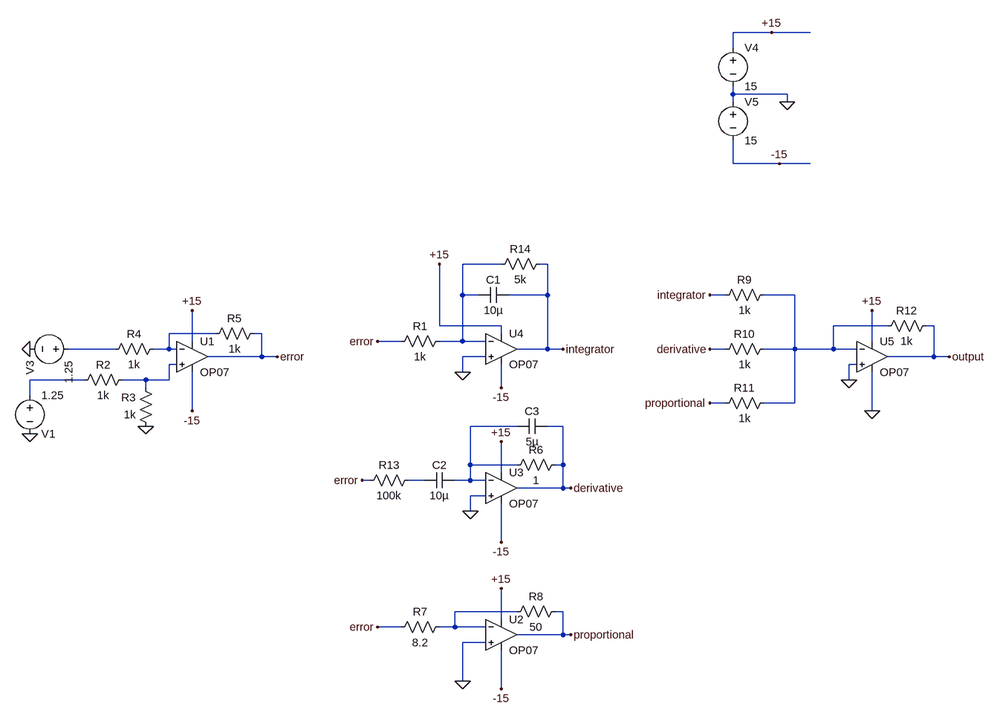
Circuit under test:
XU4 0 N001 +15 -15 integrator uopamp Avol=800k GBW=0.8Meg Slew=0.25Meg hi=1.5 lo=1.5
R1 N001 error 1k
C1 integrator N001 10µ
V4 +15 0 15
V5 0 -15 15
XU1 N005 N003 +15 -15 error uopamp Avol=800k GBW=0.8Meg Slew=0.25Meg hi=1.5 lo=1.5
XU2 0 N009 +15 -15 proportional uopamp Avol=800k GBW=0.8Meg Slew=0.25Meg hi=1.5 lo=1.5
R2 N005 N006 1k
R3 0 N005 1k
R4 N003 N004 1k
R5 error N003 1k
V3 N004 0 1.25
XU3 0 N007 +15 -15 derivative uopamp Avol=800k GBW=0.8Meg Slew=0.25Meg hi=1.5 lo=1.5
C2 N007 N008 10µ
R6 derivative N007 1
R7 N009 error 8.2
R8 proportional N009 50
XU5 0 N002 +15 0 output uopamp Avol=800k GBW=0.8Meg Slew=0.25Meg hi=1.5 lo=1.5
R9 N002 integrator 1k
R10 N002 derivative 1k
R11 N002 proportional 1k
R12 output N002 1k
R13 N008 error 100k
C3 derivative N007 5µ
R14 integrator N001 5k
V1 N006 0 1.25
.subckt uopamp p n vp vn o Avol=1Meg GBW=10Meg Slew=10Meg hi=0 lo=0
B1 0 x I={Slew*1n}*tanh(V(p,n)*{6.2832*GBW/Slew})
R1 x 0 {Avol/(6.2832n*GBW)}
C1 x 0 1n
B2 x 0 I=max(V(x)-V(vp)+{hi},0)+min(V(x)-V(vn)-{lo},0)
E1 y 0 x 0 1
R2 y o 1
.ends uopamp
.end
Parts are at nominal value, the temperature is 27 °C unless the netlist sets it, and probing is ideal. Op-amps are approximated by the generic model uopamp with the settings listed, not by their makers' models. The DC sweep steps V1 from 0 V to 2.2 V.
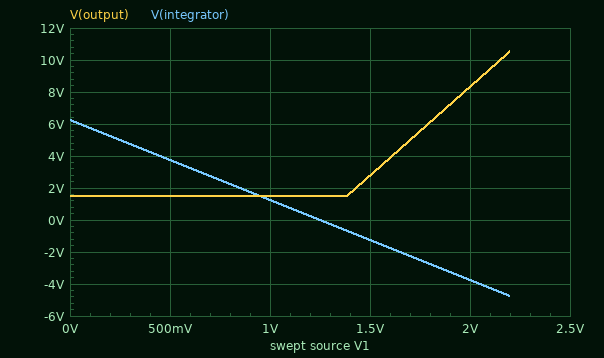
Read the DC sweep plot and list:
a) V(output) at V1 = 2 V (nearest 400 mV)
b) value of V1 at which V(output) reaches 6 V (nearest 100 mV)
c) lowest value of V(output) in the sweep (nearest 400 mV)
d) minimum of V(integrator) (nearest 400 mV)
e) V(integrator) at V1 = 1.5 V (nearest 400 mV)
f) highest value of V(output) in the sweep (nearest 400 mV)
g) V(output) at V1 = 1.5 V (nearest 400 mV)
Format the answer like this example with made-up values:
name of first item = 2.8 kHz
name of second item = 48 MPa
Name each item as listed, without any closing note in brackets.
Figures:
V(output) at V1 = 2 V = 8.4 V
value of V1 at which V(output) reaches 6 V = 1.8 V
lowest value of V(output) in the sweep = 1.6 V
minimum of V(integrator) = -4.8 V
V(integrator) at V1 = 1.5 V = -1.2 V
highest value of V(output) in the sweep = 10.4 V
V(output) at V1 = 1.5 V = 2.8 V
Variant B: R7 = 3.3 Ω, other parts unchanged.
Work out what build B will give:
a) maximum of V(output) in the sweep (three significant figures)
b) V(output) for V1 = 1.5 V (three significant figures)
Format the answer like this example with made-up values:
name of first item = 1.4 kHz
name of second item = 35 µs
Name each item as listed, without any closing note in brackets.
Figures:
maximum of V(output) in the sweep = 13.5 V
V(output) for V1 = 1.5 V = 5.04 V
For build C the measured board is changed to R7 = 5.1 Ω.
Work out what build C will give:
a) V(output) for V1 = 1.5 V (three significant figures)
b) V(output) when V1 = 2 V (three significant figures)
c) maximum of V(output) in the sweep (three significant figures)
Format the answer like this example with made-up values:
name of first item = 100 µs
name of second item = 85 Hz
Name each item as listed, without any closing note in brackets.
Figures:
V(output) for V1 = 1.5 V = 3.70 V
V(output) when V1 = 2 V = 11.1 V
maximum of V(output) in the sweep = 13.5 V
